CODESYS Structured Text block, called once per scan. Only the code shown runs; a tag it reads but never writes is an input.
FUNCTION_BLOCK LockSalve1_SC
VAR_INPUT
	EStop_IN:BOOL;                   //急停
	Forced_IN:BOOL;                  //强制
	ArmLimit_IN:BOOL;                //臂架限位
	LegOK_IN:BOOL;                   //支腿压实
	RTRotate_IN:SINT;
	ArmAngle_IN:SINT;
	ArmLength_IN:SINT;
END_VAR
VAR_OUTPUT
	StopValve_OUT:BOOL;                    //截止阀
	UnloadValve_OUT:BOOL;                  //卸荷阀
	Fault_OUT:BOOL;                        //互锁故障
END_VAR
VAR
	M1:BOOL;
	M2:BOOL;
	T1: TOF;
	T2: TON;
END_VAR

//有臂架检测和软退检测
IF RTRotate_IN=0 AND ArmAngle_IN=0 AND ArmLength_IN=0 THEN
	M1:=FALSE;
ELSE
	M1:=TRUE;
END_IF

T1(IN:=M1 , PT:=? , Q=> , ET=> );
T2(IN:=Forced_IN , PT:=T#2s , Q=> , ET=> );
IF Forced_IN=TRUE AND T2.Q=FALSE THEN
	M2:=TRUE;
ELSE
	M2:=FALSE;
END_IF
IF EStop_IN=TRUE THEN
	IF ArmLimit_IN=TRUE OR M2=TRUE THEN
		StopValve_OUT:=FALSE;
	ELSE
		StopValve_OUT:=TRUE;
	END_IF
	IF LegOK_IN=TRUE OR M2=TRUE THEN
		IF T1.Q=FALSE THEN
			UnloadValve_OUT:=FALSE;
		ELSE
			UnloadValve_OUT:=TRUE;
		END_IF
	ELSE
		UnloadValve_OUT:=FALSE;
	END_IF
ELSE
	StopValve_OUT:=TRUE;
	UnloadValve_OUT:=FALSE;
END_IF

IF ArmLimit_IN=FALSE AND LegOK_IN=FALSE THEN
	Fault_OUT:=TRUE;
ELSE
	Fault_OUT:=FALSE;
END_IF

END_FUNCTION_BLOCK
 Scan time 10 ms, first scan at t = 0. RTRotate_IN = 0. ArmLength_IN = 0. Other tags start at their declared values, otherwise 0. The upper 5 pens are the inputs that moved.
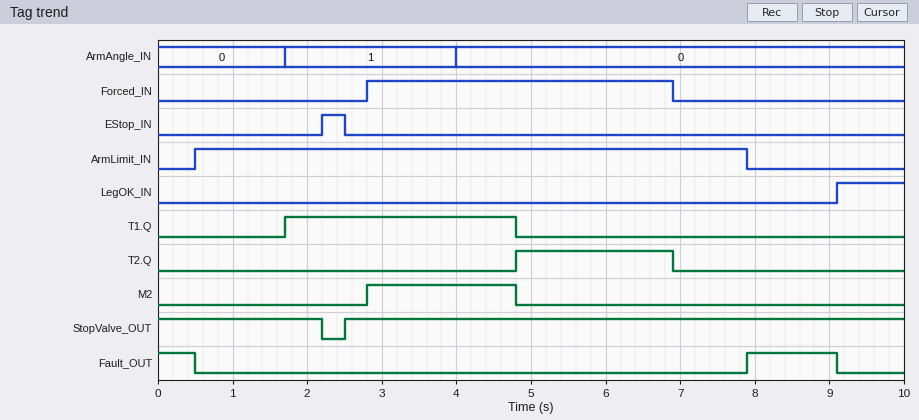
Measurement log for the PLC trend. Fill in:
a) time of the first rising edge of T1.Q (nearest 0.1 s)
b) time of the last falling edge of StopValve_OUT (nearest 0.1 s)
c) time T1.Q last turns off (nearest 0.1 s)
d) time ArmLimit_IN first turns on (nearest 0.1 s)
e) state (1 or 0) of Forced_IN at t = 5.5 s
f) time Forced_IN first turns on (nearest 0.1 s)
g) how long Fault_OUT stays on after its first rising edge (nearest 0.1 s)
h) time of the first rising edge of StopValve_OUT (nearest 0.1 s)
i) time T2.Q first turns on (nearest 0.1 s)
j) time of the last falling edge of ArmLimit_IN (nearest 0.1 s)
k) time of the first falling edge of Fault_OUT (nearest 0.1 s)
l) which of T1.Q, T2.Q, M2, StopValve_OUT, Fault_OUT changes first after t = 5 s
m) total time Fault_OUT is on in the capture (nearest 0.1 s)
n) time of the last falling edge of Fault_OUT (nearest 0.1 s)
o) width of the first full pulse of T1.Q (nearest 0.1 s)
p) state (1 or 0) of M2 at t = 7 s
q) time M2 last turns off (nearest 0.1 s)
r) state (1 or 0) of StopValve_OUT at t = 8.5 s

1.7 s
2.2 s
4.8 s
0.5 s
1
2.8 s
1.2 s
2.5 s
4.8 s
7.9 s
0.5 s
T2.Q
1.7 s
9.1 s
3.1 s
0
4.8 s
1
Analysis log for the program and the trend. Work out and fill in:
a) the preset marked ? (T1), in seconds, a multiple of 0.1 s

0.8 s
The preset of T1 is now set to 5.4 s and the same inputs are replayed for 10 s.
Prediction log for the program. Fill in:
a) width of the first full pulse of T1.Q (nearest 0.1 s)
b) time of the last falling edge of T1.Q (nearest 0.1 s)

7.7 s
9.4 s
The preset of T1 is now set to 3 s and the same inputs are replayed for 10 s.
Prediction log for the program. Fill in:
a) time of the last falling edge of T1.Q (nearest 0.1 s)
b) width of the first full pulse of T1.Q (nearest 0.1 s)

7.0 s
5.3 s
